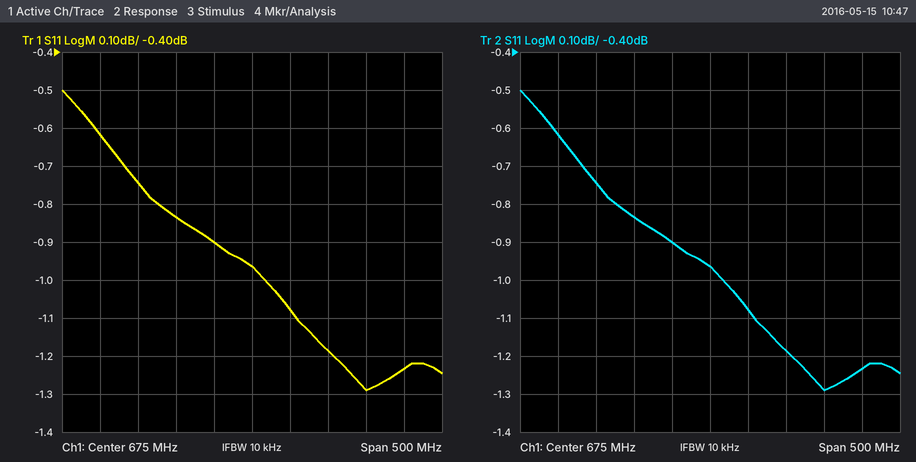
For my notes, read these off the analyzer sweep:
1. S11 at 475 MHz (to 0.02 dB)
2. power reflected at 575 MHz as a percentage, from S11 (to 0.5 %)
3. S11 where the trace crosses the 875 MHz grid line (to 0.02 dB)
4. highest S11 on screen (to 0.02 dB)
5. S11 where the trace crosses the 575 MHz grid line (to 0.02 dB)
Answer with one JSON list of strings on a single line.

["-0.62 dB", "82.5 %", "-1.24 dB", "-0.50 dB", "-0.84 dB"]
